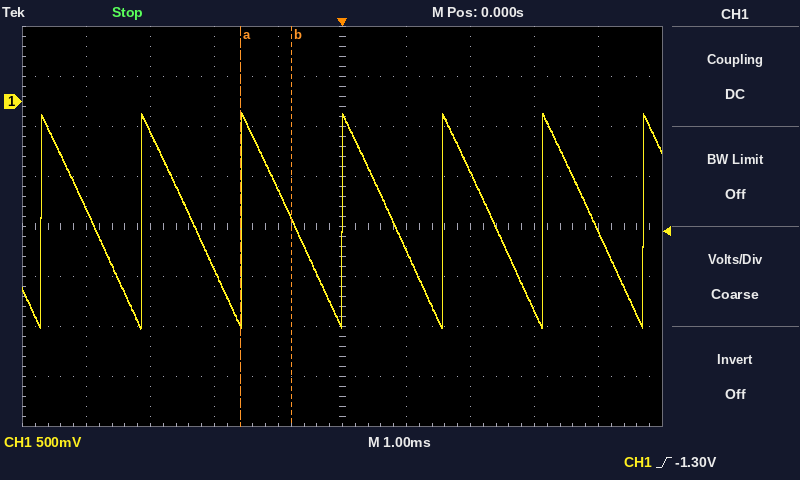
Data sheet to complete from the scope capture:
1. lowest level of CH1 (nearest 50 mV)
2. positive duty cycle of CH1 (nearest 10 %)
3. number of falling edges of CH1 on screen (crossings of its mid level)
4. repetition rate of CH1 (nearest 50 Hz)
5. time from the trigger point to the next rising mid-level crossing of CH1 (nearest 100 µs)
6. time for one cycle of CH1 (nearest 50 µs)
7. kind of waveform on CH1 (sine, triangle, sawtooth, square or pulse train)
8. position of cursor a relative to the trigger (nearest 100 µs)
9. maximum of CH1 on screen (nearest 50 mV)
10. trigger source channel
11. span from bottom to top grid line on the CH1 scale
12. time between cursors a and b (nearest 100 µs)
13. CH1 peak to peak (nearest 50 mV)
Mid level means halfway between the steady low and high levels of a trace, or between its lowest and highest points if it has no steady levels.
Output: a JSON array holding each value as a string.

["-2.25 V", "50 %", "6", "650 Hz", "1.6 ms", "1.55 ms", "sawtooth", "-1.6 ms", "-100 mV", "CH1", "4 V", "800 µs", "2.15 V"]
